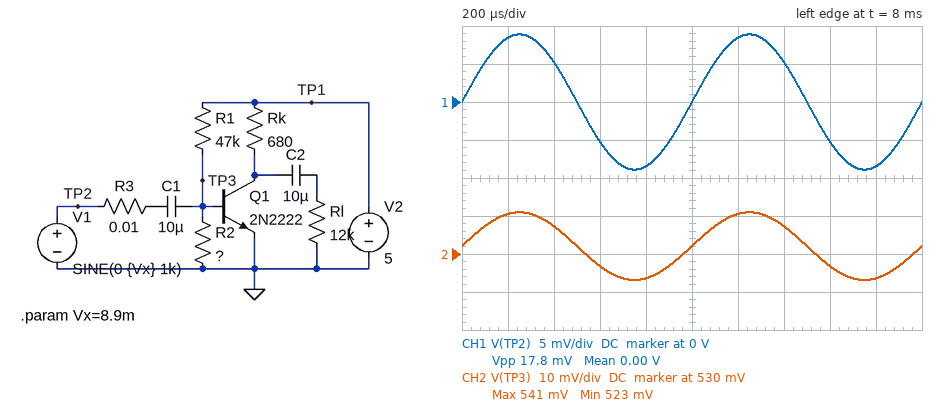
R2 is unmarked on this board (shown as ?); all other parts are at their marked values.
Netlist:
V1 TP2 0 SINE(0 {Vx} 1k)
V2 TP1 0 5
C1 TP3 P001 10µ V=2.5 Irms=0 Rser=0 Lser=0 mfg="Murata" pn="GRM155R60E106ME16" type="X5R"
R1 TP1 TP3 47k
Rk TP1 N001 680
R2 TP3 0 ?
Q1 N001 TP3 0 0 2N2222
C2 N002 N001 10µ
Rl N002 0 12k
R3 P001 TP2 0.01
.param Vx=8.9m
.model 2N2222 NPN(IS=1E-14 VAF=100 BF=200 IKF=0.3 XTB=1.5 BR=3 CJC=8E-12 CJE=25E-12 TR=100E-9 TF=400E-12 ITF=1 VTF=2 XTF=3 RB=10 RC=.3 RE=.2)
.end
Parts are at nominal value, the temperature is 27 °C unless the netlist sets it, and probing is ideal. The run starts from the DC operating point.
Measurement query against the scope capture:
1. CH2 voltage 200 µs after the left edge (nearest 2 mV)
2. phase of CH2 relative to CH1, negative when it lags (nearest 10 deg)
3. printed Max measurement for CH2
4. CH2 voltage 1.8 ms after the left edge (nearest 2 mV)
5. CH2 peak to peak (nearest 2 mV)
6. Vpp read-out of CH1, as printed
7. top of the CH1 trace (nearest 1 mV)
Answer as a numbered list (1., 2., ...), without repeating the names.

1. 540 mV
2. 0 deg
3. 541 mV
4. 524 mV
5. 18 mV
6. 17.8 mV
7. 9 mV
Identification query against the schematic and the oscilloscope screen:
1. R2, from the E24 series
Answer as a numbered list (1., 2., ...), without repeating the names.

1. 5.6 kΩ
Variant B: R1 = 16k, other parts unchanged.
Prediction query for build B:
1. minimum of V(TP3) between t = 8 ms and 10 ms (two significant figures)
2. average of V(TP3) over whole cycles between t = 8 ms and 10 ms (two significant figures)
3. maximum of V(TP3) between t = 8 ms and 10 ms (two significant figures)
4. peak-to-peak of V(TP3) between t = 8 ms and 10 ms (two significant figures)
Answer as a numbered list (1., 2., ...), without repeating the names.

1. 700 mV
2. 710 mV
3. 720 mV
4. 17 mV
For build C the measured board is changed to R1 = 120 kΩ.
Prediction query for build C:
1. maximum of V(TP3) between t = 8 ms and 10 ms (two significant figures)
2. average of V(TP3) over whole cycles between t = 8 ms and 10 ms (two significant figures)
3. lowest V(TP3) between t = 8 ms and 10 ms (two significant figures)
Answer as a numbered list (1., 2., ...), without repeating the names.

1. 230 mV
2. 220 mV
3. 210 mV
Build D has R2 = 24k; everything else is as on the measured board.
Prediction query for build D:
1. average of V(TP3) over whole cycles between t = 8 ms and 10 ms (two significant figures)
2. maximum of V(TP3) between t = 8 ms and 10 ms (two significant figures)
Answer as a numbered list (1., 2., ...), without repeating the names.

1. 700 mV
2. 710 mV
